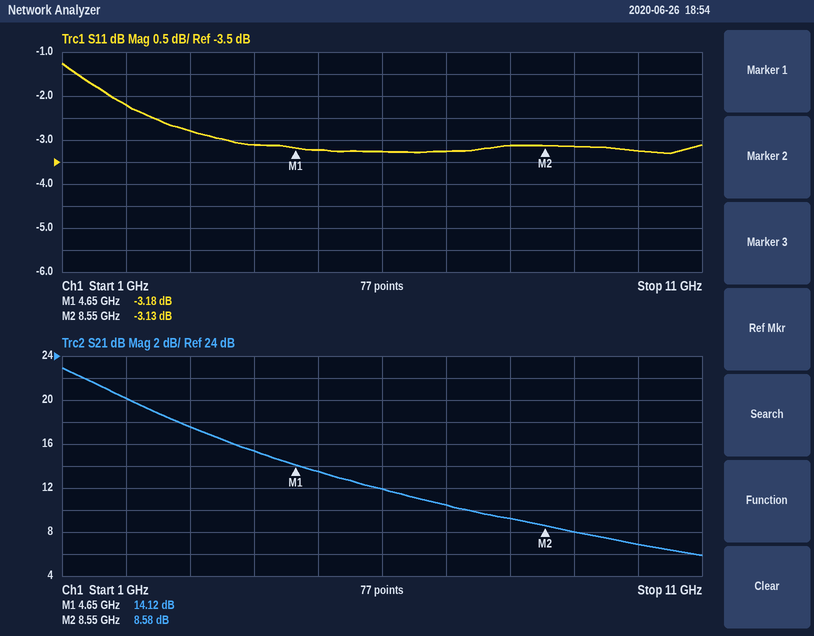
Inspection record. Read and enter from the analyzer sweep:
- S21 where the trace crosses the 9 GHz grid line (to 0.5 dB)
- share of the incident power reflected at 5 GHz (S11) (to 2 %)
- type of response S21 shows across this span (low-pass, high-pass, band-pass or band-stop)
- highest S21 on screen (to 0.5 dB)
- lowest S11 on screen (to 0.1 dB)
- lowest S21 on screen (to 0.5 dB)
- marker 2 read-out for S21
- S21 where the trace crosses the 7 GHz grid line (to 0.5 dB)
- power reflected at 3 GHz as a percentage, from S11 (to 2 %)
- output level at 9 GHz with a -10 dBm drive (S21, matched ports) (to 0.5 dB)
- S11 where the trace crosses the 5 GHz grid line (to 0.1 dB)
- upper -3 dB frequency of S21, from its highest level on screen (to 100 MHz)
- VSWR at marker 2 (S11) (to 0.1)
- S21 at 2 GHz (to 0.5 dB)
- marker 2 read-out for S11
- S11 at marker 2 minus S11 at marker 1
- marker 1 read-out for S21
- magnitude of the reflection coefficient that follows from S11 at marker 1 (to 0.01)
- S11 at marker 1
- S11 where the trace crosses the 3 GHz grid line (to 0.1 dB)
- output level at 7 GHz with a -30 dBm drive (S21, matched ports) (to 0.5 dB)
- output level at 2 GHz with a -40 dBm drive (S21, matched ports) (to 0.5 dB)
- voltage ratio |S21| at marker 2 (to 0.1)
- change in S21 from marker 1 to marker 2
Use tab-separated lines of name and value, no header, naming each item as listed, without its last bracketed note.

S21 where the trace crosses the 9 GHz grid line	8.0 dB
share of the incident power reflected at 5 GHz (S11)	48 %
type of response S21 shows across this span	low-pass
highest S21 on screen	23.0 dB
lowest S11 on screen	-3.3 dB
lowest S21 on screen	6.0 dB
marker 2 read-out for S21	8.58 dB
S21 where the trace crosses the 7 GHz grid line	10.5 dB
power reflected at 3 GHz as a percentage, from S11	52 %
output level at 9 GHz with a -10 dBm drive (S21, matched ports)	-2.0 dBm
S11 where the trace crosses the 5 GHz grid line	-3.2 dB
upper -3 dB frequency of S21, from its highest level on screen	2.1 GHz
VSWR at marker 2 (S11)	5.6
S21 at 2 GHz	20.0 dB
marker 2 read-out for S11	-3.13 dB
S11 at marker 2 minus S11 at marker 1	0.05 dB
marker 1 read-out for S21	14.12 dB
magnitude of the reflection coefficient that follows from S11 at marker 1	0.69
S11 at marker 1	-3.18 dB
S11 where the trace crosses the 3 GHz grid line	-2.8 dB
output level at 7 GHz with a -30 dBm drive (S21, matched ports)	-19.5 dBm
output level at 2 GHz with a -40 dBm drive (S21, matched ports)	-20.0 dBm
voltage ratio |S21| at marker 2	2.7
change in S21 from marker 1 to marker 2	-5.54 dB
